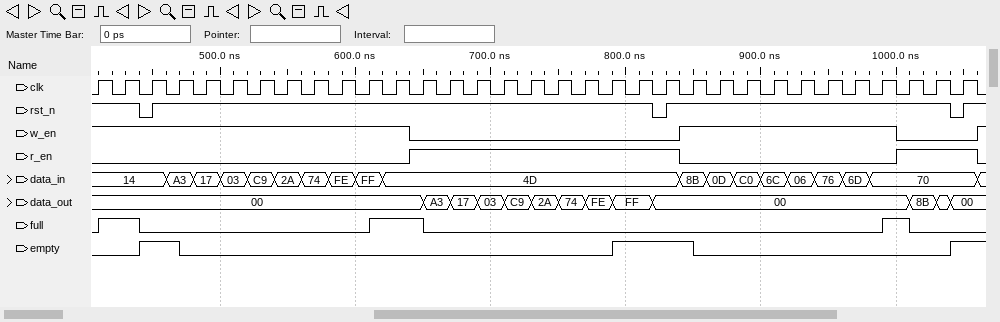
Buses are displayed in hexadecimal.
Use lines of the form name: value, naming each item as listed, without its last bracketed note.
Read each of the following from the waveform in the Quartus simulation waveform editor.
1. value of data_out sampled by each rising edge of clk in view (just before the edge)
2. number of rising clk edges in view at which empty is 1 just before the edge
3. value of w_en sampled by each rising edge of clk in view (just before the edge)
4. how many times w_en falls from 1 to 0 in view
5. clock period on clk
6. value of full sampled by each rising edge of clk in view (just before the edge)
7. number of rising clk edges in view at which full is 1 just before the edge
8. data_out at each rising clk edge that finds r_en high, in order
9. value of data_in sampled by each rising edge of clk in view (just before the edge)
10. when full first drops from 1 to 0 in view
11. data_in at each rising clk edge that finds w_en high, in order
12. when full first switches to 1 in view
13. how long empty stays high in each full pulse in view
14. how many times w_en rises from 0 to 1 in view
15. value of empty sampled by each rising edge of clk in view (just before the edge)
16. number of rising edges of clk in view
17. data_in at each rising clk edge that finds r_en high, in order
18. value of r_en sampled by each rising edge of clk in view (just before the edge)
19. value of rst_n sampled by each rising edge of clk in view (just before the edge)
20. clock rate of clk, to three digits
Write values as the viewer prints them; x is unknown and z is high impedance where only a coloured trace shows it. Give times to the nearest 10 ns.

value of data_out sampled by each rising edge of clk in view: 00, 00, 00, 00, 00, 00, 00, 00, 00, 00, 00, 00, 00, A3, 17, 03, C9, 2A, 74, FE, FF, 00, 00, 00, 00, 00, 00, 00, 00, 00, 00, 8B, 00
number of rising clk edges in view at which empty is 1 just before the edge: 6
value of w_en sampled by each rising edge of clk in view: 1 1 1 1 1 1 1 1 1 1 1 1 0 0 0 0 0 0 0 0 0 0 1 1 1 1 1 1 1 1 0 0 0
how many times w_en falls from 1 to 0 in view: 2
clock period on clk: 20 ns
value of full sampled by each rising edge of clk in view: 0 1 0 0 0 0 0 0 0 0 0 1 1 0 0 0 0 0 0 0 0 0 0 0 0 0 0 0 0 0 1 0 0
number of rising clk edges in view at which full is 1 just before the edge: 4
data_out at each rising clk edge that finds r_en high, in order: 00, A3, 17, 03, C9, 2A, 74, FE, FF, 00, 00, 8B, 00
value of data_in sampled by each rising edge of clk in view: 14, 14, 14, A3, 17, 03, C9, 2A, 74, FE, FF, 4D, 4D, 4D, 4D, 4D, 4D, 4D, 4D, 4D, 4D, 4D, 8B, 0D, C0, 6C, 06, 76, 6D, 70, 70, 70, 70
when full first drops from 1 to 0 in view: 440 ns
data_in at each rising clk edge that finds w_en high, in order: 14, 14, 14, A3, 17, 03, C9, 2A, 74, FE, FF, 4D, 8B, 0D, C0, 6C, 06, 76, 6D, 70
when full first switches to 1 in view: 410 ns
how long empty stays high in each full pulse in view: 30 ns, 60 ns
how many times w_en rises from 0 to 1 in view: 2
value of empty sampled by each rising edge of clk in view: 0 0 1 1 0 0 0 0 0 0 0 0 0 0 0 0 0 0 0 0 1 1 1 0 0 0 0 0 0 0 0 0 1
number of rising edges of clk in view: 33
data_in at each rising clk edge that finds r_en high, in order: 4D, 4D, 4D, 4D, 4D, 4D, 4D, 4D, 4D, 4D, 70, 70, 70
value of r_en sampled by each rising edge of clk in view: 0 0 0 0 0 0 0 0 0 0 0 0 1 1 1 1 1 1 1 1 1 1 0 0 0 0 0 0 0 0 1 1 1
value of rst_n sampled by each rising edge of clk in view: 1 1 0 1 1 1 1 1 1 1 1 1 1 1 1 1 1 1 1 1 1 0 1 1 1 1 1 1 1 1 1 1 0
clock rate of clk, to three digits: 50.0 MHz
